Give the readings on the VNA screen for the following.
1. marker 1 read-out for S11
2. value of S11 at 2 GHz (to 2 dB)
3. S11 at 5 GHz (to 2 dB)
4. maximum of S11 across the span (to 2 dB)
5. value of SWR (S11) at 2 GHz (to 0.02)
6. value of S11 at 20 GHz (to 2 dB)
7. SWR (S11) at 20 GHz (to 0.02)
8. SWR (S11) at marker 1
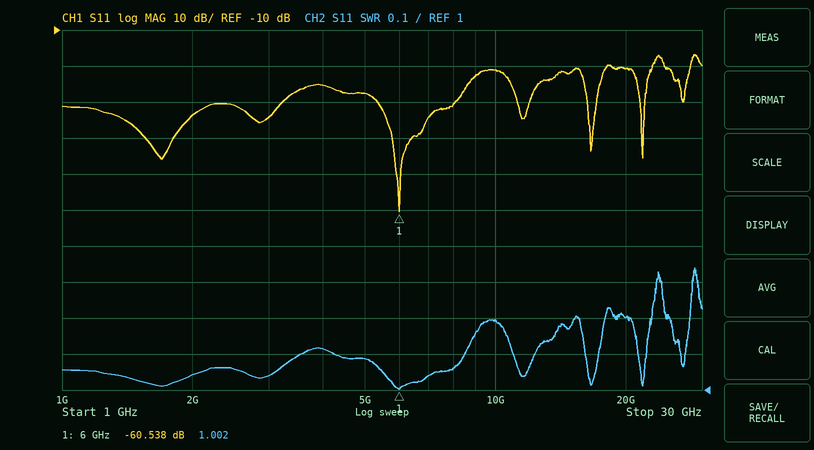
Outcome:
-60.538 dB
-34 dB
-28 dB
-16 dB
1.04
-20 dB
1.20
1.002
